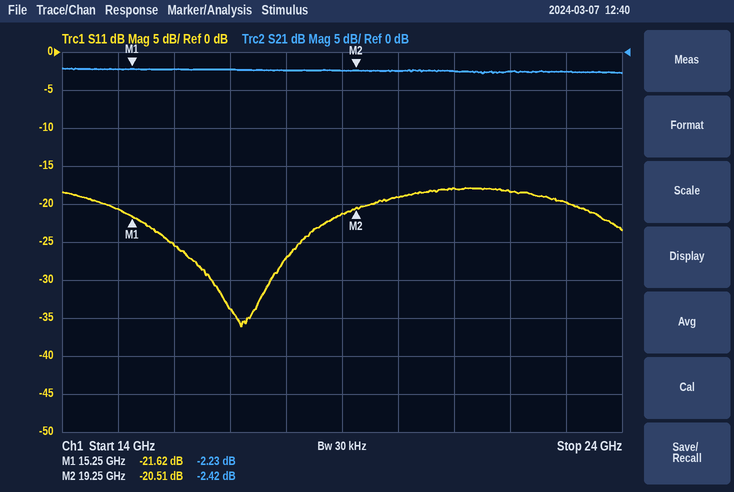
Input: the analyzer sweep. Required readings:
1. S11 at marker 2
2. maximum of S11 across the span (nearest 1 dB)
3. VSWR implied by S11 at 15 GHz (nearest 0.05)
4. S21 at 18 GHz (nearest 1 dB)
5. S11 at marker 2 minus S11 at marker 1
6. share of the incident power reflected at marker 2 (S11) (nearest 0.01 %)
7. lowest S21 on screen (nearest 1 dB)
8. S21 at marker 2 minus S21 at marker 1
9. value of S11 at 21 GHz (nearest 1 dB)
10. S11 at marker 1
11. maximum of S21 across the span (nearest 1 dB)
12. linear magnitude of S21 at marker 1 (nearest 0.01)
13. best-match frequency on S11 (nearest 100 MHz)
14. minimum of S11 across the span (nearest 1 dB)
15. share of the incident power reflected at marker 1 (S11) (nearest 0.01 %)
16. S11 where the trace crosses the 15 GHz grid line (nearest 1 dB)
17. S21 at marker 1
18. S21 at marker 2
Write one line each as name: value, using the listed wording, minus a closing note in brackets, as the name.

S11 at marker 2: -20.51 dB
maximum of S11 across the span: -18 dB
VSWR implied by S11 at 15 GHz: 1.20
S21 at 18 GHz: -2 dB
S11 at marker 2 minus S11 at marker 1: 1.11 dB
share of the incident power reflected at marker 2 (S11): 0.89 %
lowest S21 on screen: -3 dB
S21 at marker 2 minus S21 at marker 1: -0.19 dB
value of S11 at 21 GHz: -18 dB
S11 at marker 1: -21.62 dB
maximum of S21 across the span: -2 dB
linear magnitude of S21 at marker 1: 0.77
best-match frequency on S11: 17.2 GHz
minimum of S11 across the span: -36 dB
share of the incident power reflected at marker 1 (S11): 0.69 %
S11 where the trace crosses the 15 GHz grid line: -21 dB
S21 at marker 1: -2.23 dB
S21 at marker 2: -2.42 dB
